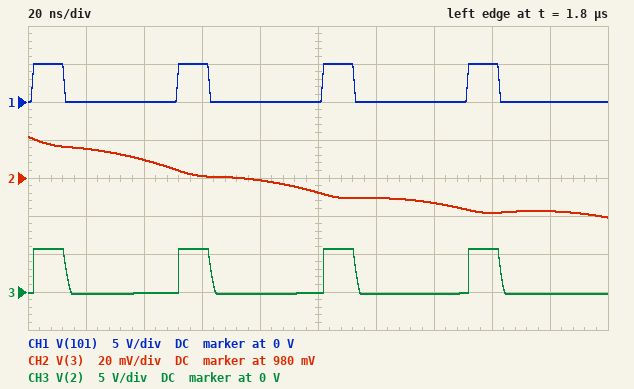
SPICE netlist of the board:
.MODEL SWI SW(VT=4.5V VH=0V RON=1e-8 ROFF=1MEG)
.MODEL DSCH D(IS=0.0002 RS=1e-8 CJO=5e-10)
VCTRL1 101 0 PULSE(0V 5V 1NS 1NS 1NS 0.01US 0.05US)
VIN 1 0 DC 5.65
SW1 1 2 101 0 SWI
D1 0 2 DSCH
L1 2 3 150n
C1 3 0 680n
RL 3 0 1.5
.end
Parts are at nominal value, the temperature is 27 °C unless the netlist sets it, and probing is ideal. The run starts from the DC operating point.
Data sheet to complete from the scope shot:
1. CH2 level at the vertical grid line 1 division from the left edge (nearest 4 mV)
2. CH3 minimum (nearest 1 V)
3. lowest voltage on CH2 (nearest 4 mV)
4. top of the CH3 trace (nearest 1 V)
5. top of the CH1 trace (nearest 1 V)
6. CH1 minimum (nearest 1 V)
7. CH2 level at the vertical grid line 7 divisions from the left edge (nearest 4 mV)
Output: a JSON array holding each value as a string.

["996 mV", "0 V", "960 mV", "6 V", "5 V", "0 V", "968 mV"]
